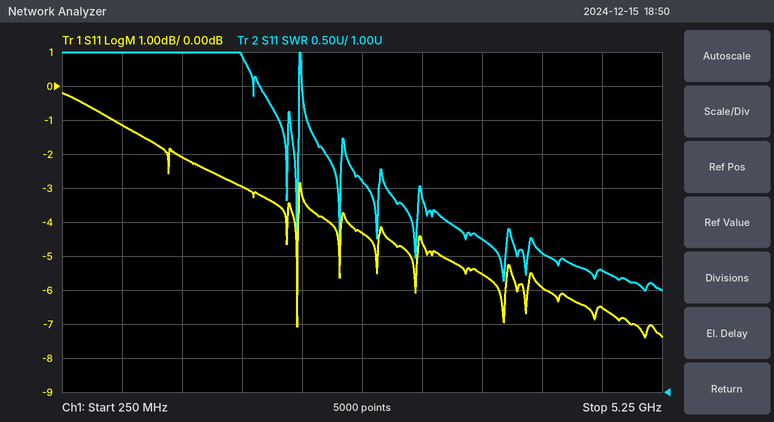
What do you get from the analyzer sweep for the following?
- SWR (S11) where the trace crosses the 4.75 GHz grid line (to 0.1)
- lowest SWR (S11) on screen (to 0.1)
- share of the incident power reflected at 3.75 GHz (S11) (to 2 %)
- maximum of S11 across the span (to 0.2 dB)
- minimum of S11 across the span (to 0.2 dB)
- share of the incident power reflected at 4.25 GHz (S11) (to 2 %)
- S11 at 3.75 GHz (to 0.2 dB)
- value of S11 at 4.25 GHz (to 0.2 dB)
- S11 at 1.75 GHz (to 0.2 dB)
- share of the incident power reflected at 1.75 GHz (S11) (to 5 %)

2.8
2.5
28 %
-0.2 dB
-7.4 dB
26 %
-5.6 dB
-6.0 dB
-3.0 dB
50 %
